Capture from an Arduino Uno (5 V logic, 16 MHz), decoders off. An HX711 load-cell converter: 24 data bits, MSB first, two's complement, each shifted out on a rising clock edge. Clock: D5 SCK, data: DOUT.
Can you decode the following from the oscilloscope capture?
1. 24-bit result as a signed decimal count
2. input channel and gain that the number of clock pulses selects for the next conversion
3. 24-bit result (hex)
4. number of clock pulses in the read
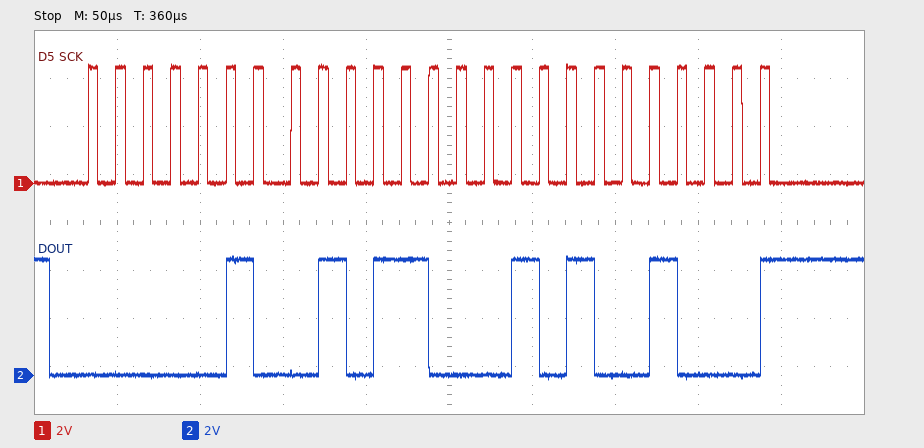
307528
channel A, gain 128
0x04B148
25
